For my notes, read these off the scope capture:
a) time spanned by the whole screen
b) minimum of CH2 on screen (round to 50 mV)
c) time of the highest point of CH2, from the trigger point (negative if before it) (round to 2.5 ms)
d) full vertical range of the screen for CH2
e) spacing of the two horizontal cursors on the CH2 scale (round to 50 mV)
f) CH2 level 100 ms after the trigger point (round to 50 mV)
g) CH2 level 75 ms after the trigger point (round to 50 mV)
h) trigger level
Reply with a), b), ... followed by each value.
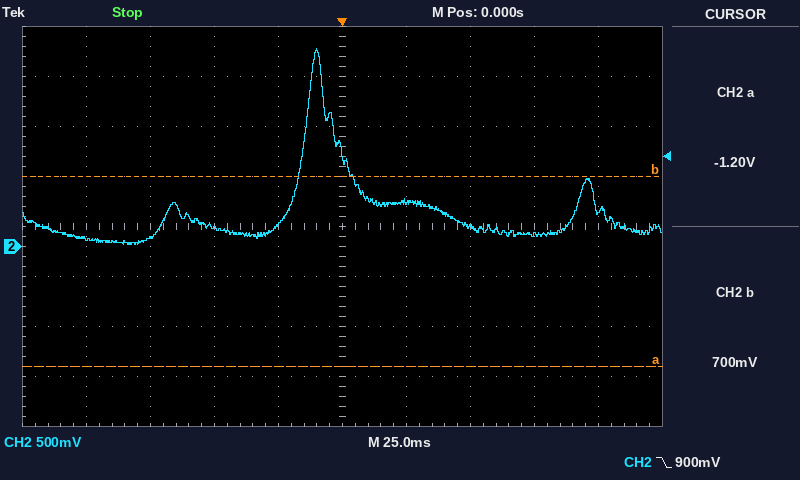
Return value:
a) 250 ms
b) 0 mV
c) -10.0 ms
d) 4 V
e) 1.90 V
f) 350 mV
g) 100 mV
h) 900 mV
